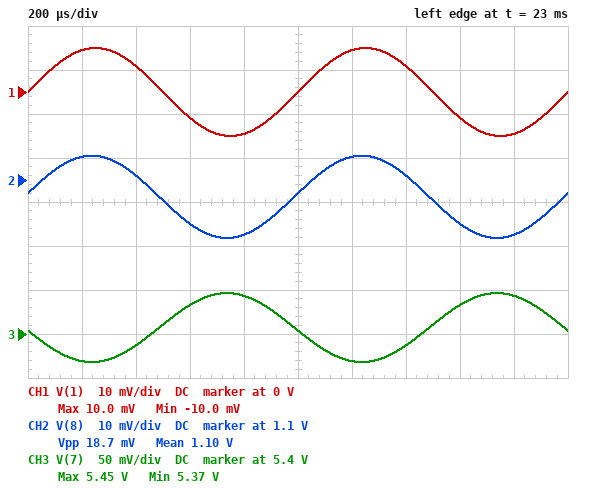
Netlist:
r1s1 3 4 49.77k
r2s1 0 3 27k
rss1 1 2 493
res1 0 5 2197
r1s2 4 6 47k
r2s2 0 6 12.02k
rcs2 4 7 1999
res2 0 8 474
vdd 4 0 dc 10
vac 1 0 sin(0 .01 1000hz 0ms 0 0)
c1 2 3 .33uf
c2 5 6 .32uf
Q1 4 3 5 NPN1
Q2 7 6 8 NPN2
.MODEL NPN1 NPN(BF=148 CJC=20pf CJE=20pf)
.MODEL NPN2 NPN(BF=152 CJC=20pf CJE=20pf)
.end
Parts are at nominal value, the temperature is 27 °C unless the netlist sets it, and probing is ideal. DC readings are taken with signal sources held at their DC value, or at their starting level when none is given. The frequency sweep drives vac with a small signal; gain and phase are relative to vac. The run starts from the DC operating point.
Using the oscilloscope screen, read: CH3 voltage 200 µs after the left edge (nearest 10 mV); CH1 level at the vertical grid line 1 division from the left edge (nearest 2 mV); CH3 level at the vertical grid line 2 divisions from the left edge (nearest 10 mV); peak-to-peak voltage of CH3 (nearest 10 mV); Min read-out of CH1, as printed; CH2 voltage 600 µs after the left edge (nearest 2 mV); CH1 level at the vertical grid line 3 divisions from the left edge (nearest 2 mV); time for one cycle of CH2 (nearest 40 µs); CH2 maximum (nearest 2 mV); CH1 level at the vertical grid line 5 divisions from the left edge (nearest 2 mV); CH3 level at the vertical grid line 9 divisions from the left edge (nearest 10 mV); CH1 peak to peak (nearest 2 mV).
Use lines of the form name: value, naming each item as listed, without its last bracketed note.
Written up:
CH3 voltage 200 µs after the left edge: 5.37 V
CH1 level at the vertical grid line 1 division from the left edge: 10 mV
CH3 level at the vertical grid line 2 divisions from the left edge: 5.39 V
peak-to-peak voltage of CH3: 80 mV
Min read-out of CH1, as printed: -10.0 mV
CH2 voltage 600 µs after the left edge: 1.090 V
CH1 level at the vertical grid line 3 divisions from the left edge: -6 mV
time for one cycle of CH2: 1.00 ms
CH2 maximum: 1.106 V
CH1 level at the vertical grid line 5 divisions from the left edge: 0 V
CH3 level at the vertical grid line 9 divisions from the left edge: 5.44 V
CH1 peak to peak: 20 mV
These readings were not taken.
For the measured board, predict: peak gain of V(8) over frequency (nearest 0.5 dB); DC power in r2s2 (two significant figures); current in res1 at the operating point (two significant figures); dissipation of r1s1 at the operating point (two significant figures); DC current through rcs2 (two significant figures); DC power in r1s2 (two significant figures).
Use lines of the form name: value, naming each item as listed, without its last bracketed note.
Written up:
peak gain of V(8) over frequency: -0.5 dB
DC power in r2s2: 300 µW
current in res1 at the operating point: 1.2 mA
dissipation of r1s1 at the operating point: 880 µW
DC current through rcs2: 2.3 mA
DC power in r1s2: 1.4 mW
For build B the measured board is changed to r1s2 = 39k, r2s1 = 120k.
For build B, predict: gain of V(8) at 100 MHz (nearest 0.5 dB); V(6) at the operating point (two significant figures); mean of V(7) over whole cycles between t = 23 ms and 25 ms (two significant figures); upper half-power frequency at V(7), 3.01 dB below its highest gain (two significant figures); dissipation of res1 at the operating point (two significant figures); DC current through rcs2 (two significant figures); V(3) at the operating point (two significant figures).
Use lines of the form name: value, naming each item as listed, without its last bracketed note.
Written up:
gain of V(8) at 100 MHz: -12.5 dB
V(6) at the operating point: 2.2 V
mean of V(7) over whole cycles between t = 23 ms and 25 ms: 4.2 V
upper half-power frequency at V(7), 3.01 dB below its highest gain: 6.1 MHz
dissipation of res1 at the operating point: 15 mW
DC current through rcs2: 2.9 mA
V(3) at the operating point: 6.5 V
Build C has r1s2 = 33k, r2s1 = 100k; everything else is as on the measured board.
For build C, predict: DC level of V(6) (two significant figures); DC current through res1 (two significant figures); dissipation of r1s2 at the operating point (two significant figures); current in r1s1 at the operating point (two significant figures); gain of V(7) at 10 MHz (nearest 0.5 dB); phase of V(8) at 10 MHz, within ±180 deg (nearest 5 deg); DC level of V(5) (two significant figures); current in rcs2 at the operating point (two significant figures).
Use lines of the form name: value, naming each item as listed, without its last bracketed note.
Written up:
DC level of V(6): 2.5 V
DC current through res1: 2.4 mA
dissipation of r1s2 at the operating point: 1.7 mW
current in r1s1 at the operating point: 78 µA
gain of V(7) at 10 MHz: 5.0 dB
phase of V(8) at 10 MHz, within ±180 deg: -20 deg
DC level of V(5): 5.3 V
current in rcs2 at the operating point: 3.5 mA
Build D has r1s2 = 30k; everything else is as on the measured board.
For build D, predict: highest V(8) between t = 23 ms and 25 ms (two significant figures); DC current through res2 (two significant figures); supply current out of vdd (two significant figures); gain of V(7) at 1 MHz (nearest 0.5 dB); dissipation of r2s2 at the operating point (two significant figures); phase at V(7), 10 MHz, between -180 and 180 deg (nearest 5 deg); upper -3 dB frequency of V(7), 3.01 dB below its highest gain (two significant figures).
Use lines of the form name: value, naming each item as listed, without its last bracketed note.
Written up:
highest V(8) between t = 23 ms and 25 ms: 1.8 V
DC current through res2: 3.9 mA
supply current out of vdd: 5.4 mA
gain of V(7) at 1 MHz: 11.5 dB
dissipation of r2s2 at the operating point: 580 µW
phase at V(7), 10 MHz, between -180 and 180 deg: 50 deg
upper -3 dB frequency of V(7), 3.01 dB below its highest gain: 3.3 MHz
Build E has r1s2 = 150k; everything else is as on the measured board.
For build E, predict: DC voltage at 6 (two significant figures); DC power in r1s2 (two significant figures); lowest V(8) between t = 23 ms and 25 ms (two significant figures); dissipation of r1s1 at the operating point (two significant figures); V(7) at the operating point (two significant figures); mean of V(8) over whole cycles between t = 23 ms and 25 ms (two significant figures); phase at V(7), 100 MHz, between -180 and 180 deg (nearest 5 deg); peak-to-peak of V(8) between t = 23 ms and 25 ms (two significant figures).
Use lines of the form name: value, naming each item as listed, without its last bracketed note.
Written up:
DC voltage at 6: 740 mV
DC power in r1s2: 570 µW
lowest V(8) between t = 23 ms and 25 ms: 27 mV
dissipation of r1s1 at the operating point: 880 µW
V(7) at the operating point: 9.9 V
mean of V(8) over whole cycles between t = 23 ms and 25 ms: 32 mV
phase at V(7), 100 MHz, between -180 and 180 deg: -65 deg
peak-to-peak of V(8) between t = 23 ms and 25 ms: 11 mV
